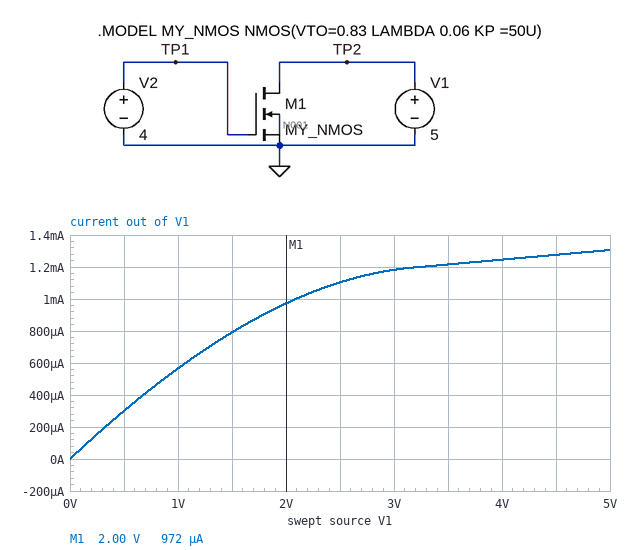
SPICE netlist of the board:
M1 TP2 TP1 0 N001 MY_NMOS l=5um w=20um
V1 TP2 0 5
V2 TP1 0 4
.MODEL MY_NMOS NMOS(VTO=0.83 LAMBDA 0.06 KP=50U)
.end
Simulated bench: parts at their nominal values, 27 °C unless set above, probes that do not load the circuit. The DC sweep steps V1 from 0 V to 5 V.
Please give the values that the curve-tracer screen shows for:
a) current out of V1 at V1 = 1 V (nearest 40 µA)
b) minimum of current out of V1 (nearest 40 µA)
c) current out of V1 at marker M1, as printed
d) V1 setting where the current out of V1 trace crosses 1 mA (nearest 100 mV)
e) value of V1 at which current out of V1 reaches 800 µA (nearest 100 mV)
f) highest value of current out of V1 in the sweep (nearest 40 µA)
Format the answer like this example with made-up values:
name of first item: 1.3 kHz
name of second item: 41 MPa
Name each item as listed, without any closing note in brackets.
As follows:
current out of V1 at V1 = 1 V: 560 µA
minimum of current out of V1: 0 A
current out of V1 at marker M1, as printed: 972 µA
V1 setting where the current out of V1 trace crosses 1 mA: 2.1 V
value of V1 at which current out of V1 reaches 800 µA: 1.5 V
highest value of current out of V1 in the sweep: 1.32 mA
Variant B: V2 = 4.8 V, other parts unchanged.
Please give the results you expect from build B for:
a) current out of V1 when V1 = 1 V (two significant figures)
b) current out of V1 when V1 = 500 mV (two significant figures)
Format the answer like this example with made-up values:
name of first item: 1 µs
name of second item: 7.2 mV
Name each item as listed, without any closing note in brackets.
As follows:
current out of V1 when V1 = 1 V: 740 µA
current out of V1 when V1 = 500 mV: 380 µA
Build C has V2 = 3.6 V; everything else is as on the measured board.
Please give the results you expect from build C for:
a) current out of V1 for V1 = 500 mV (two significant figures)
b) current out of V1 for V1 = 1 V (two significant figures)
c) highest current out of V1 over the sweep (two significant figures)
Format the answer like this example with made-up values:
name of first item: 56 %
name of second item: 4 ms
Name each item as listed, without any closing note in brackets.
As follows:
current out of V1 for V1 = 500 mV: 260 µA
current out of V1 for V1 = 1 V: 480 µA
highest current out of V1 over the sweep: 1.0 mA
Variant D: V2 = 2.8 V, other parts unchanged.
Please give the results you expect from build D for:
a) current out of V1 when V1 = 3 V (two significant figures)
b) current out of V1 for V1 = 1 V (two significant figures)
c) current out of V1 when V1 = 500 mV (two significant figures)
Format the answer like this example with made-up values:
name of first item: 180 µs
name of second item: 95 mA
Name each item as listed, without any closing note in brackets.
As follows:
current out of V1 when V1 = 3 V: 460 µA
current out of V1 for V1 = 1 V: 310 µA
current out of V1 when V1 = 500 mV: 180 µA
